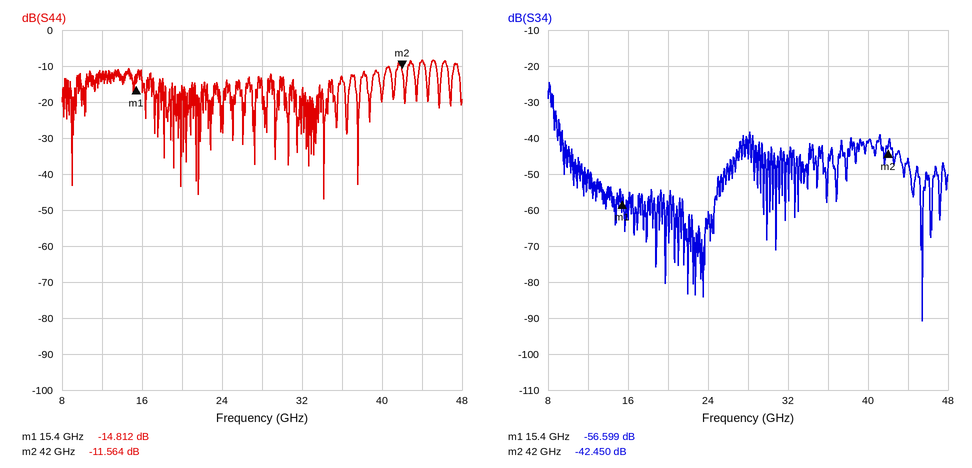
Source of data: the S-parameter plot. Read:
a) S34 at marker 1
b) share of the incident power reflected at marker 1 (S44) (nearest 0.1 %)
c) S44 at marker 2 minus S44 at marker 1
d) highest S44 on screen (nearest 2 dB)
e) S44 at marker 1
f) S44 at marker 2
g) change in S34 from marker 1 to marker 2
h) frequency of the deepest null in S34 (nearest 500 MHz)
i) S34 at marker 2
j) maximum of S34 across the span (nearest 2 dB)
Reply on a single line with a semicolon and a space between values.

-56.599 dB; 3.3 %; 3.248 dB; -8 dB; -14.812 dB; -11.564 dB; 14.149 dB; 45.5 GHz; -42.450 dB; -24 dB
